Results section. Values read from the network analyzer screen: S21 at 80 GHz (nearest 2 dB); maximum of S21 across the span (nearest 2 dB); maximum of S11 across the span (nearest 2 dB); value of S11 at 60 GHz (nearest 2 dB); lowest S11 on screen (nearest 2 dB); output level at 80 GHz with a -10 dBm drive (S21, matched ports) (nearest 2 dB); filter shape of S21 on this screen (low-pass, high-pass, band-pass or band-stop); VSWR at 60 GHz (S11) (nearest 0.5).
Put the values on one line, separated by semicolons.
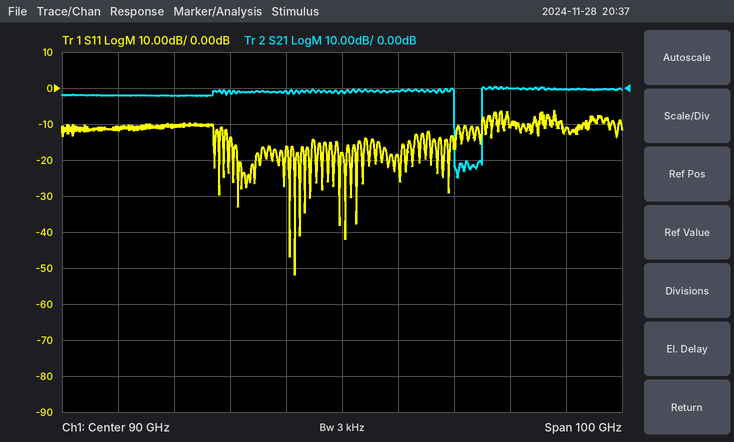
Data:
0 dB; 0 dB; -6 dB; -10 dB; -52 dB; -10 dBm; band-stop; 2.0
